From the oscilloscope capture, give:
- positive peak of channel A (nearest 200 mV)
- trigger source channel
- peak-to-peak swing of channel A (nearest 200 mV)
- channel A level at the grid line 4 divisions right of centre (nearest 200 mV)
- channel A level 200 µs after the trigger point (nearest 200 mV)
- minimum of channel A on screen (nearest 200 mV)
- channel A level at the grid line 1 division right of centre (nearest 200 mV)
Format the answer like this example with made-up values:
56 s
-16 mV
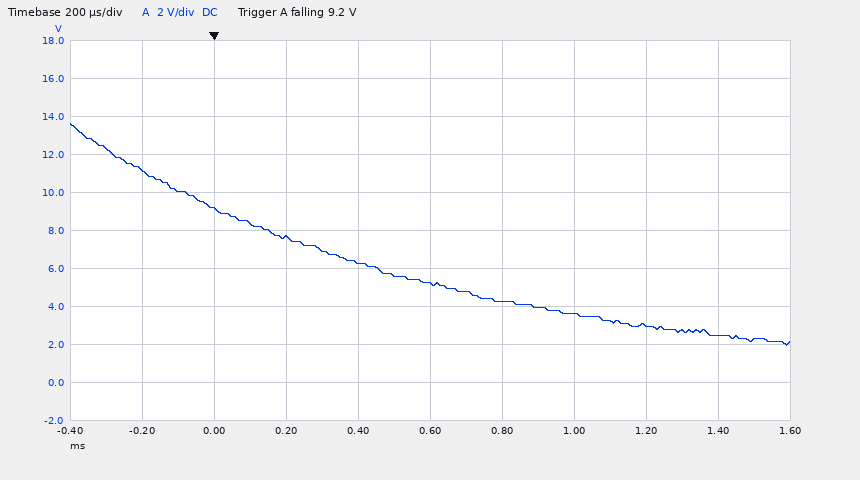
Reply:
13.6 V
channel A
11.6 V
2.4 V
7.6 V
2.0 V
4.2 V
